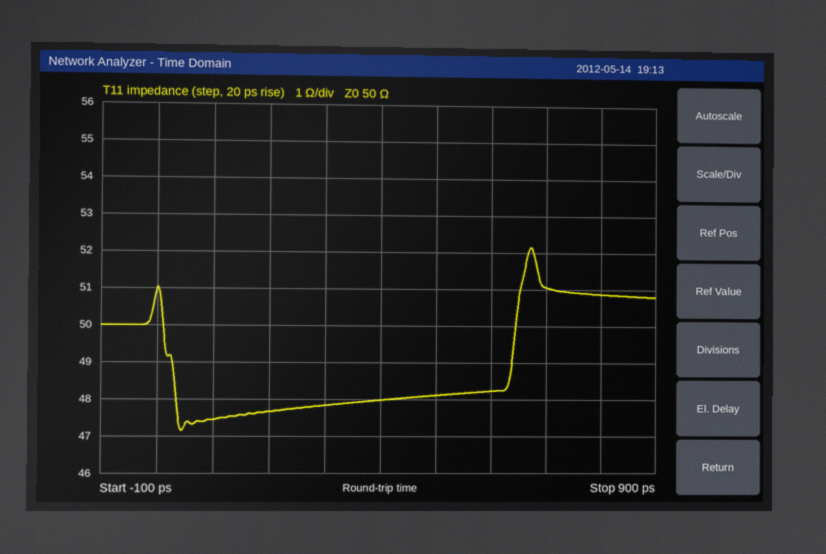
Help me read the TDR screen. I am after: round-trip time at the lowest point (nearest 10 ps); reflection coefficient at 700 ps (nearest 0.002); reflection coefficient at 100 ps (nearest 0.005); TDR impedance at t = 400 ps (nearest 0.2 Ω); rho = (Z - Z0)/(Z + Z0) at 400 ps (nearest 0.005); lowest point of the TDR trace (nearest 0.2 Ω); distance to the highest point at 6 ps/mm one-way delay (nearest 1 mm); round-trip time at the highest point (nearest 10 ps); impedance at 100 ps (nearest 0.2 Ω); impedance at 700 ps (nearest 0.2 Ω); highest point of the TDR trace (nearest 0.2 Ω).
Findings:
40 ps
+0.010
-0.025
48.0 Ω
-0.020
47.2 Ω
56 mm
670 ps
47.4 Ω
51.0 Ω
52.2 Ω
